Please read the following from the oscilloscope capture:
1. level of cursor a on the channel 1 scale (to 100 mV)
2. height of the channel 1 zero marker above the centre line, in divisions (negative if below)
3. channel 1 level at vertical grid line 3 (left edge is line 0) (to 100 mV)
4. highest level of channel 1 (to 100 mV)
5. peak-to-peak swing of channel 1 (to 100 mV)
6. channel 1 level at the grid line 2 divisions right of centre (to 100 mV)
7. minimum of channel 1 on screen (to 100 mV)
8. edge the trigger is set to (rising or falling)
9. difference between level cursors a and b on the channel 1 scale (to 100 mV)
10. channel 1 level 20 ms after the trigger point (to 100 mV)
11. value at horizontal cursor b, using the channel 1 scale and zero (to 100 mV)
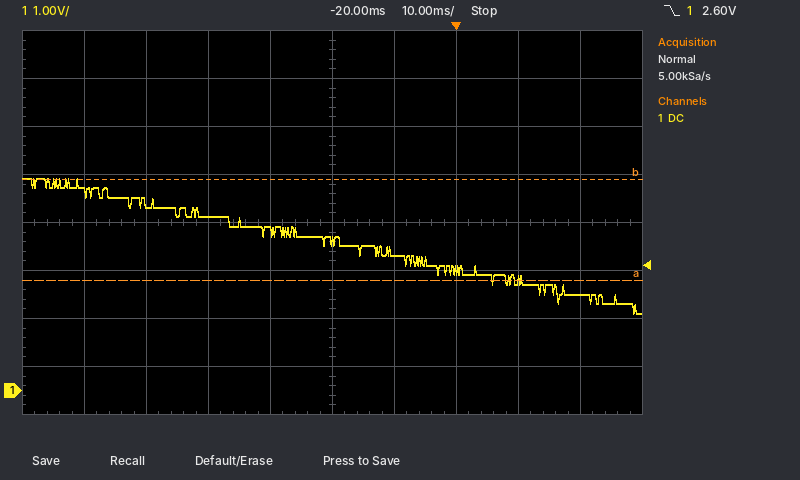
2.3 V
-3.5 div
3.6 V
4.4 V
2.8 V
2.5 V
1.6 V
falling
2.1 V
2.0 V
4.4 V
